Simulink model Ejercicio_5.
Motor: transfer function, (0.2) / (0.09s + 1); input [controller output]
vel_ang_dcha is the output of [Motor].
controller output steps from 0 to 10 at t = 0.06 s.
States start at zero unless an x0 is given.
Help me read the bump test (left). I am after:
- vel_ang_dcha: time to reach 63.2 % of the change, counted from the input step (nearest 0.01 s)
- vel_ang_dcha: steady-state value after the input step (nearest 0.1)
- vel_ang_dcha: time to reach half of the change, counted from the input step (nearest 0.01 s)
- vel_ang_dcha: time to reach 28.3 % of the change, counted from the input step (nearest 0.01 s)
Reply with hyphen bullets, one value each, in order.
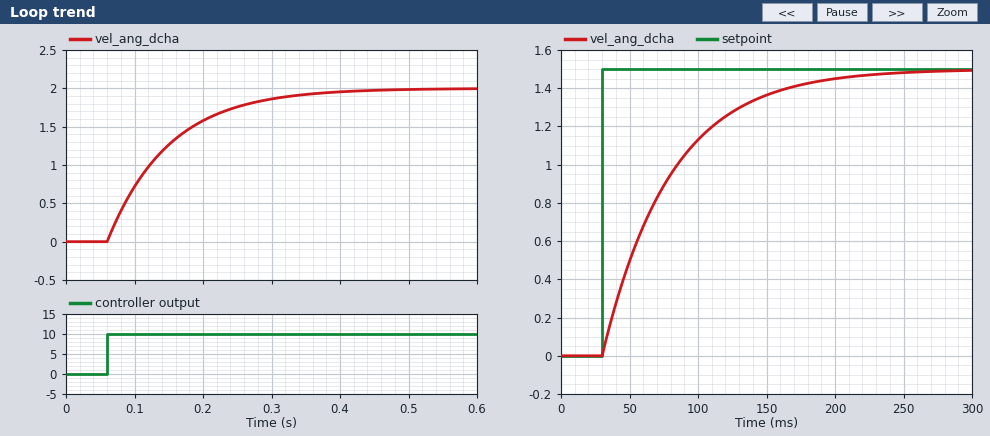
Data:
- 0.09 s
- 2.0
- 0.06 s
- 0.03 s
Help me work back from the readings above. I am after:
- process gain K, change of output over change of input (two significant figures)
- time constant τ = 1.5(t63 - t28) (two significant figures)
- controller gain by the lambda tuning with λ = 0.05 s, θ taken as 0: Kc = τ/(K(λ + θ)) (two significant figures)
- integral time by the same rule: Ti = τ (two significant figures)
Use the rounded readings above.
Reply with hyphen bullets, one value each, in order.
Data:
- 0.20
- 0.090 s
- 9.0
- 0.090 s
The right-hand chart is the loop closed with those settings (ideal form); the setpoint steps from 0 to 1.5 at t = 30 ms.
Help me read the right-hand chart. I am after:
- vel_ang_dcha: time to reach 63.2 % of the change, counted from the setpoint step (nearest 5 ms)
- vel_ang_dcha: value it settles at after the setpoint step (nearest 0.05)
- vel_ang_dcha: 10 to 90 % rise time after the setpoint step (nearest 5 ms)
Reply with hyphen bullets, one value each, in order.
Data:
- 50 ms
- 1.50
- 110 ms
